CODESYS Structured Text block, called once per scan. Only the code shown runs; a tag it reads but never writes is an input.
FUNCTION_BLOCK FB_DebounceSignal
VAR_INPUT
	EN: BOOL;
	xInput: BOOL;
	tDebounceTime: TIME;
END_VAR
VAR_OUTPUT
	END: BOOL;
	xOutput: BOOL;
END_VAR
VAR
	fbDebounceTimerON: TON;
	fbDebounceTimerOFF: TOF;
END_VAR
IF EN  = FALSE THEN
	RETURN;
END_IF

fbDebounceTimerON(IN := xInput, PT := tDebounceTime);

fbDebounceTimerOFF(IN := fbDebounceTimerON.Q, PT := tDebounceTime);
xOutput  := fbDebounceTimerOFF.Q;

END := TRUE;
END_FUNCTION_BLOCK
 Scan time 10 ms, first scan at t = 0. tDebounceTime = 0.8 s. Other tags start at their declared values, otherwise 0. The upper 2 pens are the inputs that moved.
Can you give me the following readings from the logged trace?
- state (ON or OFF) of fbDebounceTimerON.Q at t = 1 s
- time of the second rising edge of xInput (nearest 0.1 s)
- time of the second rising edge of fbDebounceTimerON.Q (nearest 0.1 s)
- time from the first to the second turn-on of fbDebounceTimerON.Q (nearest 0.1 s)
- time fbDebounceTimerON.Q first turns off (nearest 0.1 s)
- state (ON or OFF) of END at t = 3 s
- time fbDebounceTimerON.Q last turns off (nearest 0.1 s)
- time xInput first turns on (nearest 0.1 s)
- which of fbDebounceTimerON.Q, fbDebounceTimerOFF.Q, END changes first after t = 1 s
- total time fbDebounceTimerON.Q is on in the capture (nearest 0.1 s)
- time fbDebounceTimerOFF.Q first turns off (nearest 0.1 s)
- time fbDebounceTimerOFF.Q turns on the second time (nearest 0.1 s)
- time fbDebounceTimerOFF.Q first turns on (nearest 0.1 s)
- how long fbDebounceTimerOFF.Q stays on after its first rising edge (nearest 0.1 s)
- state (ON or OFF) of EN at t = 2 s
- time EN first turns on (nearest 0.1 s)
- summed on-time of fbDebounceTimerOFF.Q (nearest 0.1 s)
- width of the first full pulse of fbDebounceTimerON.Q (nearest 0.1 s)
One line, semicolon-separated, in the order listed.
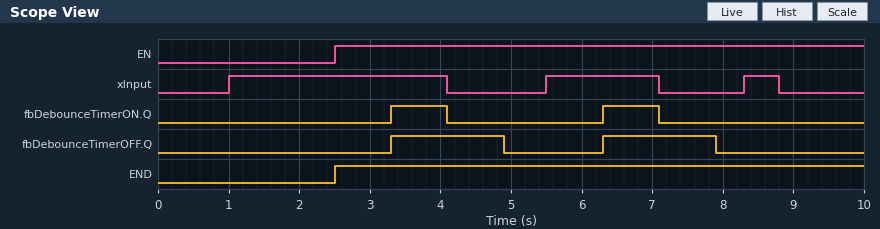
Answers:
OFF; 5.5 s; 6.3 s; 3.0 s; 4.1 s; ON; 7.1 s; 1.0 s; END; 1.6 s; 4.9 s; 6.3 s; 3.3 s; 1.6 s; OFF; 2.5 s; 3.2 s; 0.8 s
